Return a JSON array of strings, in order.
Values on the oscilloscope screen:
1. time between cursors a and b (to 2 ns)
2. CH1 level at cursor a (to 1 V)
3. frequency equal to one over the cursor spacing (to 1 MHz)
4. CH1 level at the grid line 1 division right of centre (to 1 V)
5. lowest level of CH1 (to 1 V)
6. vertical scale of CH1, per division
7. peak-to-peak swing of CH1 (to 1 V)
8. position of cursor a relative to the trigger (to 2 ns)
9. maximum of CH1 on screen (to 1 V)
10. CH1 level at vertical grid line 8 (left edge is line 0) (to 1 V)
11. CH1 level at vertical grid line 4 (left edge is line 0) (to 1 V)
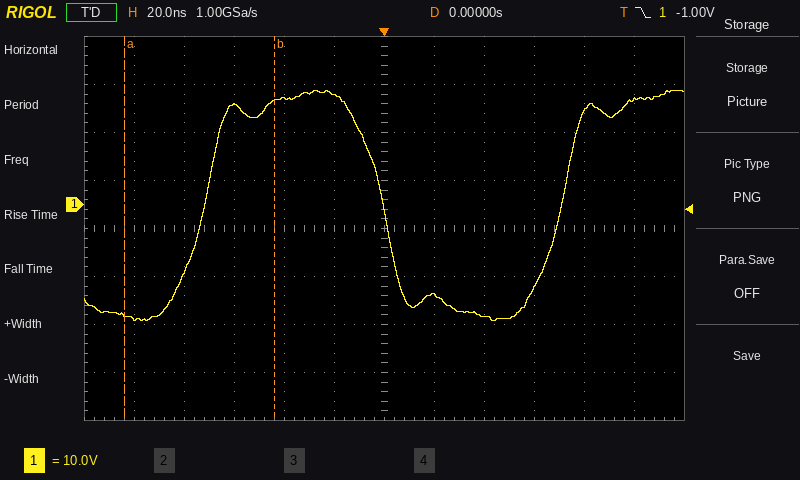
["60 ns", "-23 V", "17 MHz", "-19 V", "-24 V", "10 V", "48 V", "-104 ns", "24 V", "-23 V", "22 V"]
